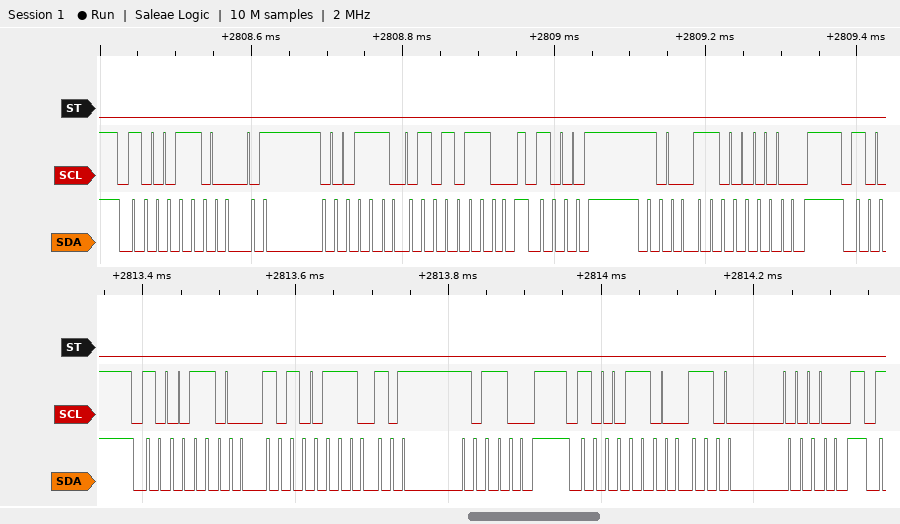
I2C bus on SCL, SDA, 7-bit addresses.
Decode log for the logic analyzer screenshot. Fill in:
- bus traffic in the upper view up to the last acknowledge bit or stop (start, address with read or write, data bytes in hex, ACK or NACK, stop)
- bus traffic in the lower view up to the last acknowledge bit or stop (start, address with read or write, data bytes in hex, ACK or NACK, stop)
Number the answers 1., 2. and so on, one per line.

1. start, address 46 write ACK, 47 ACK, 56 ACK, stop, start, address 46 write ACK, C0 ACK, stop
2. start, address 46 write ACK, A7 ACK, B6 ACK, stop, start, address 46 write ACK, C0 ACK, stop
